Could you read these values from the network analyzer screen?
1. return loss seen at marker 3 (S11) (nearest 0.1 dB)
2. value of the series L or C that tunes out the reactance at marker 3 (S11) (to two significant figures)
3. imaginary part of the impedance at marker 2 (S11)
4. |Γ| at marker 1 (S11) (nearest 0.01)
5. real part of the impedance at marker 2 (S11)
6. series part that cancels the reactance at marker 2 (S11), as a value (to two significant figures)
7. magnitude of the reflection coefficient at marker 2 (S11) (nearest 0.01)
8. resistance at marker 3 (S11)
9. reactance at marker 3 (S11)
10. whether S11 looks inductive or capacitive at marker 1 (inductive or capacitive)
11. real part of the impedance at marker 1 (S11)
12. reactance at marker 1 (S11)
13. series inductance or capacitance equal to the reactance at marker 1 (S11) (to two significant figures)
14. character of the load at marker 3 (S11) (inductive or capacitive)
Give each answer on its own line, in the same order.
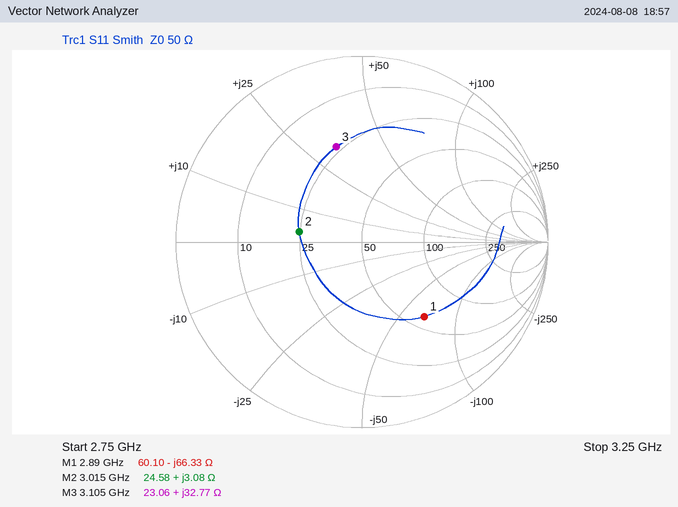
5.5 dB
1.6 pF
+3.08 Ω
0.52
24.58 Ω
17 pF
0.34
23.06 Ω
+32.77 Ω
capacitive
60.10 Ω
-66.33 Ω
830 fF
inductive
